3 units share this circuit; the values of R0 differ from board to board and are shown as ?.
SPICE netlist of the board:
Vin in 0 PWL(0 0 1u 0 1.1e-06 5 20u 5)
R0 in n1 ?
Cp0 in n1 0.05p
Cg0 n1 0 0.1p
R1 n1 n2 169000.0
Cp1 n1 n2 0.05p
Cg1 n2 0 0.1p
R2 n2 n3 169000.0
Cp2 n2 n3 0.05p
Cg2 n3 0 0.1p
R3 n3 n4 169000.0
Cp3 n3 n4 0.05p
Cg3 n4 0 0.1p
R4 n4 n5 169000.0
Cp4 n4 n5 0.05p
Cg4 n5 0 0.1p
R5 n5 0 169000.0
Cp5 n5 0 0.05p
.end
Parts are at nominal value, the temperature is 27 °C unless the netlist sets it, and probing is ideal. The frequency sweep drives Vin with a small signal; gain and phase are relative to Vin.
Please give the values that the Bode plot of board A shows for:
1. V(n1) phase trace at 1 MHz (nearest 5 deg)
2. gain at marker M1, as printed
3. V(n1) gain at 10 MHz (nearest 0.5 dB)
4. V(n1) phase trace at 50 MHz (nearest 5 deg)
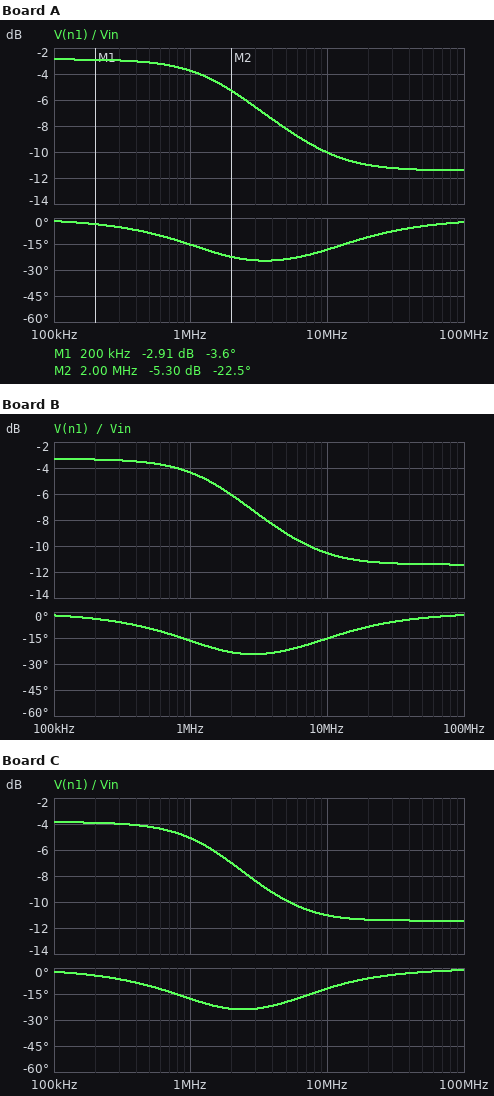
-15 deg
-2.91 dB
-10.0 dB
-5 deg
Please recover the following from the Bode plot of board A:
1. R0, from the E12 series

330 kΩ
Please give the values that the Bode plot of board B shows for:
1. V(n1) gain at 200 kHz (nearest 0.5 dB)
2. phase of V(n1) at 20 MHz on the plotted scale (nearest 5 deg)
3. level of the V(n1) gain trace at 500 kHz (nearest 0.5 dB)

-3.5 dB
-10 deg
-3.5 dB
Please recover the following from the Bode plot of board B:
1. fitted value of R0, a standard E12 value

390 kΩ
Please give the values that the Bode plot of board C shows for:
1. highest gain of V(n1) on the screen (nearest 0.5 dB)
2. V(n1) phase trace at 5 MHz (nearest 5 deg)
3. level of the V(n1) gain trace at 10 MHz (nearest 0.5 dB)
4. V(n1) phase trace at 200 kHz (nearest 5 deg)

-4.0 dB
-20 deg
-11.0 dB
-5 deg
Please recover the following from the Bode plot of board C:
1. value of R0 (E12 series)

470 kΩ
